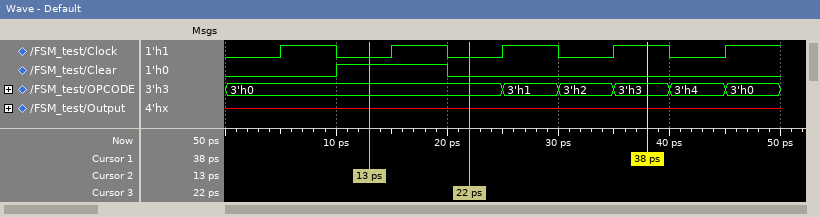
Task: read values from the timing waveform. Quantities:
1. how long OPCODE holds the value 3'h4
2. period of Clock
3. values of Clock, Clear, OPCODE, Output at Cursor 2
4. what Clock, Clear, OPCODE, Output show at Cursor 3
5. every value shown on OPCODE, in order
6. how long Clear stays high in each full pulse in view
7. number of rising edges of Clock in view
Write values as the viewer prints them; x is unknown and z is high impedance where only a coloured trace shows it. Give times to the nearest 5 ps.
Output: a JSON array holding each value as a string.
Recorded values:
["5 ps", "10 ps", "Clock=0, Clear=1, OPCODE=3'h0, Output=x", "Clock=0, Clear=0, OPCODE=3'h0, Output=x", "3'h0, 3'h1, 3'h2, 3'h3, 3'h4, 3'h0", "10 ps", "5"]
